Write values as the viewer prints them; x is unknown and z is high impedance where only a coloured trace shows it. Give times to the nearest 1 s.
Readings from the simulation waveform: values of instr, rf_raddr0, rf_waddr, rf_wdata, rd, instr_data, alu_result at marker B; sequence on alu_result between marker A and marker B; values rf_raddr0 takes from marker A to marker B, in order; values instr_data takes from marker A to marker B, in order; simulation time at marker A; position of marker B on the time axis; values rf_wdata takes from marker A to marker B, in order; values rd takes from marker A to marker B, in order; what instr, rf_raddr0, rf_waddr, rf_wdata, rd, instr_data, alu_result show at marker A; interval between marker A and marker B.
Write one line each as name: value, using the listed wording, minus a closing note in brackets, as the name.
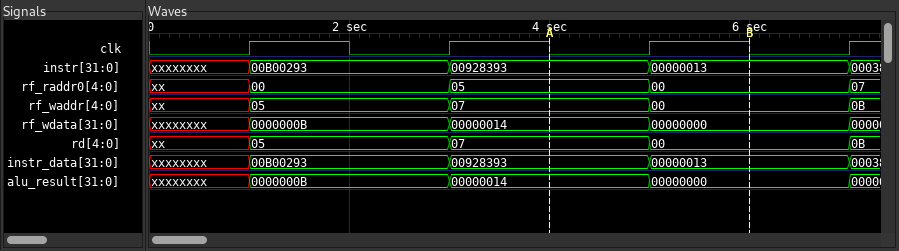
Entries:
values of instr, rf_raddr0, rf_waddr, rf_wdata, rd, instr_data, alu_result at marker B: instr=00000013, rf_raddr0=00, rf_waddr=00, rf_wdata=00000000, rd=00, instr_data=00000013, alu_result=00000000
sequence on alu_result between marker A and marker B: 00000014, 00000000
values rf_raddr0 takes from marker A to marker B, in order: 05, 00
values instr_data takes from marker A to marker B, in order: 00928393, 00000013
simulation time at marker A: 4 s
position of marker B on the time axis: 6 s
values rf_wdata takes from marker A to marker B, in order: 00000014, 00000000
values rd takes from marker A to marker B, in order: 07, 00
what instr, rf_raddr0, rf_waddr, rf_wdata, rd, instr_data, alu_result show at marker A: instr=00928393, rf_raddr0=05, rf_waddr=07, rf_wdata=00000014, rd=07, instr_data=00928393, alu_result=00000014
interval between marker A and marker B: 2 s
